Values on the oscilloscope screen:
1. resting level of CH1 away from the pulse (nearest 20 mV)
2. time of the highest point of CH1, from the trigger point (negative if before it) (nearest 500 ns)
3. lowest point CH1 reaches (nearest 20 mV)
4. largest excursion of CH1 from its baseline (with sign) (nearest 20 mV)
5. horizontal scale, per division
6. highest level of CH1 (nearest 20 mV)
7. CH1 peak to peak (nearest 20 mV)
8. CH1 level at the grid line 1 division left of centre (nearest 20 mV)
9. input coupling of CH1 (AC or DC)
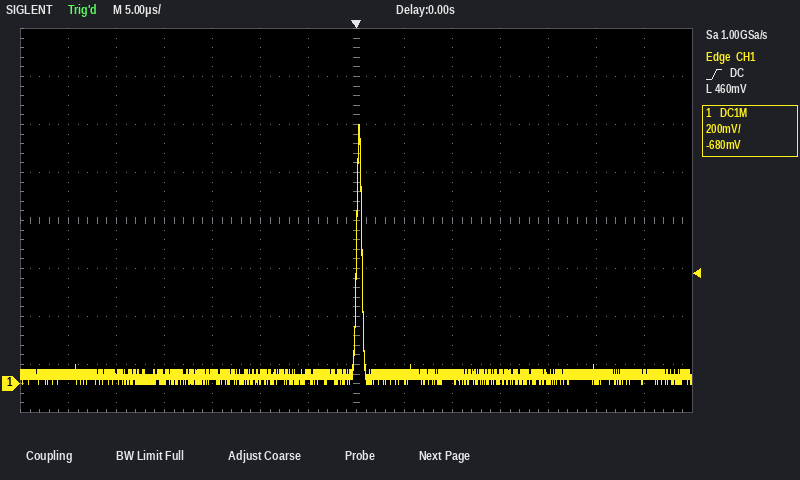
40 mV
+500 ns
0 mV
+1.04 V
5 µs
1.08 V
1.08 V
40 mV
DC
